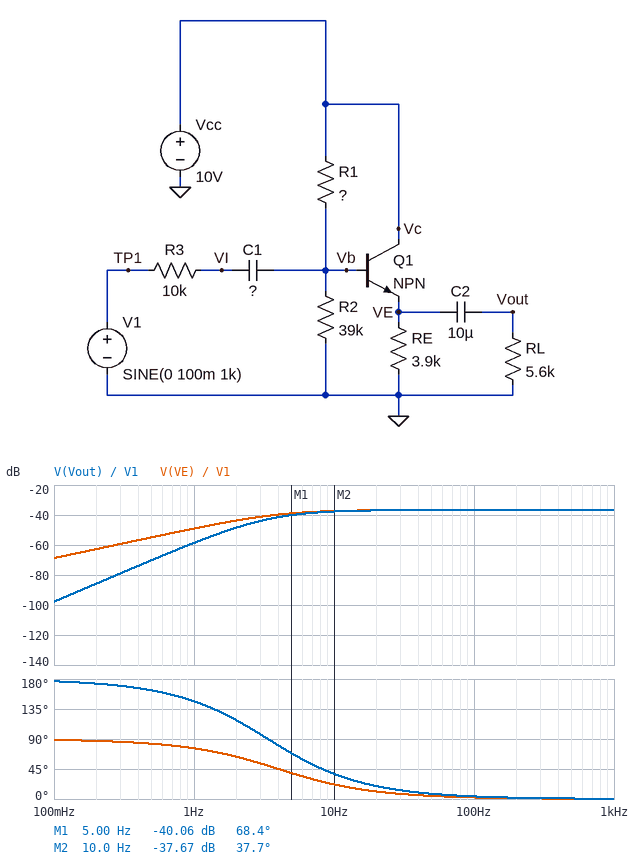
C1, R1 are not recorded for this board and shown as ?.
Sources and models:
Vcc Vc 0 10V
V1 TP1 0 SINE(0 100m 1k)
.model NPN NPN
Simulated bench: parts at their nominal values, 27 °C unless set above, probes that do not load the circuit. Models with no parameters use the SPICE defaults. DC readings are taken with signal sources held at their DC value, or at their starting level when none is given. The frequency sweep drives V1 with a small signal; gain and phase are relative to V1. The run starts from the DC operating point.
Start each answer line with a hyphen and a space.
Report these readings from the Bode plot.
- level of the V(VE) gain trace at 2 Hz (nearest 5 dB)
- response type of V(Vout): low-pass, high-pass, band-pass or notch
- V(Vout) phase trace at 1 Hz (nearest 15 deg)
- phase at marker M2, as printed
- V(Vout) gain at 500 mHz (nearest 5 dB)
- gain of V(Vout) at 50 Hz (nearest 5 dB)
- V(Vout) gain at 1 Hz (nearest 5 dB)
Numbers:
- -45 dB
- high-pass
- 150 deg
- 37.7 deg
- -70 dB
- -35 dB
- -60 dB
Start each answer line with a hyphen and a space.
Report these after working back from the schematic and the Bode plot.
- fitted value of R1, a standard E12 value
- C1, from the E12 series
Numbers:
- 150 Ω
- 3.9 µF
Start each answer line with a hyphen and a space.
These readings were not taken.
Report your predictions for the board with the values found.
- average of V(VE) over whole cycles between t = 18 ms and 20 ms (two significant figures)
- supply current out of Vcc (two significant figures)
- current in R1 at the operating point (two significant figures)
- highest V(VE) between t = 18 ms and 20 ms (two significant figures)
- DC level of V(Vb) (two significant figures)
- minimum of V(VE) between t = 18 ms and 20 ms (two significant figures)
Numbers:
- 9.2 V
- 2.6 mA
- 280 µA
- 9.2 V
- 10 V
- 9.2 V
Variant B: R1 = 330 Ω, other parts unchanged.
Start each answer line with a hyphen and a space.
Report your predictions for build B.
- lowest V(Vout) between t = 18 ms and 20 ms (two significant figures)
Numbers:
- -3.2 mV
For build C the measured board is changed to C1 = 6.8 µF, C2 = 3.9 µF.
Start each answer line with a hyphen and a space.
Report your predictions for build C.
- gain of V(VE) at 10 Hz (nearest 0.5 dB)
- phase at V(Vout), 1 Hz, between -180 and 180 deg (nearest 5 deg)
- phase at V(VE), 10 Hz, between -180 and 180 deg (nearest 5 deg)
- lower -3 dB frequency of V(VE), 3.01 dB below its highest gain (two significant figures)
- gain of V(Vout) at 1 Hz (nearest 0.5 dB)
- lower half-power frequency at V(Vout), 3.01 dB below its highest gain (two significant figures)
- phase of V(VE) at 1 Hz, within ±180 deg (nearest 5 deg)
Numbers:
- -37.0 dB
- 150 deg
- 15 deg
- 2.3 Hz
- -62.0 dB
- 7.9 Hz
- 65 deg
